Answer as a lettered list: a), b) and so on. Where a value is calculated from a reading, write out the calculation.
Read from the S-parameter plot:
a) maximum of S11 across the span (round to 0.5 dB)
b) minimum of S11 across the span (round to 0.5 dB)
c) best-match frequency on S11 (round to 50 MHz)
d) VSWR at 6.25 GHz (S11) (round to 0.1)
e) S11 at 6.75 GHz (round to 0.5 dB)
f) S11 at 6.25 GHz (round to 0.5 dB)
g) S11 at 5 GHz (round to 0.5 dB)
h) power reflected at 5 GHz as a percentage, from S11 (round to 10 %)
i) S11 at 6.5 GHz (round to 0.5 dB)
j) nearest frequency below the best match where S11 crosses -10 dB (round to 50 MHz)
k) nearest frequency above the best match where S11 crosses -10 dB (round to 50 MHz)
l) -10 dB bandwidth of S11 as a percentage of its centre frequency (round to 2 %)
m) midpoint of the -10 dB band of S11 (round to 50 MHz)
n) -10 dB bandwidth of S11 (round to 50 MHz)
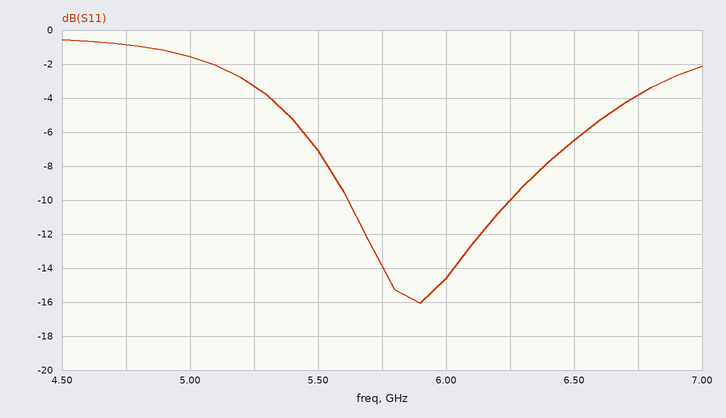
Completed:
a) -0.5 dB
b) -16.0 dB
c) 5.90 GHz
d) |Γ| = 10^(-10/20) = 0.3162; VSWR = (1 + 0.3162)/(1 − 0.3162) ≈ 1.9
e) -4.0 dB
f) -10.0 dB
g) -1.5 dB
h) 10^(-1.5/10) ≈ 70.8 %, so 70 % to the nearest 10 %
i) -6.5 dB
j) 5.60 GHz
k) 6.25 GHz
l) 650 MHz / 5.925 GHz ≈ 11.0 %, so 10 % to the nearest 2 %
m) 5.95 GHz
n) 6.25 GHz − 5.60 GHz = 650 MHz
